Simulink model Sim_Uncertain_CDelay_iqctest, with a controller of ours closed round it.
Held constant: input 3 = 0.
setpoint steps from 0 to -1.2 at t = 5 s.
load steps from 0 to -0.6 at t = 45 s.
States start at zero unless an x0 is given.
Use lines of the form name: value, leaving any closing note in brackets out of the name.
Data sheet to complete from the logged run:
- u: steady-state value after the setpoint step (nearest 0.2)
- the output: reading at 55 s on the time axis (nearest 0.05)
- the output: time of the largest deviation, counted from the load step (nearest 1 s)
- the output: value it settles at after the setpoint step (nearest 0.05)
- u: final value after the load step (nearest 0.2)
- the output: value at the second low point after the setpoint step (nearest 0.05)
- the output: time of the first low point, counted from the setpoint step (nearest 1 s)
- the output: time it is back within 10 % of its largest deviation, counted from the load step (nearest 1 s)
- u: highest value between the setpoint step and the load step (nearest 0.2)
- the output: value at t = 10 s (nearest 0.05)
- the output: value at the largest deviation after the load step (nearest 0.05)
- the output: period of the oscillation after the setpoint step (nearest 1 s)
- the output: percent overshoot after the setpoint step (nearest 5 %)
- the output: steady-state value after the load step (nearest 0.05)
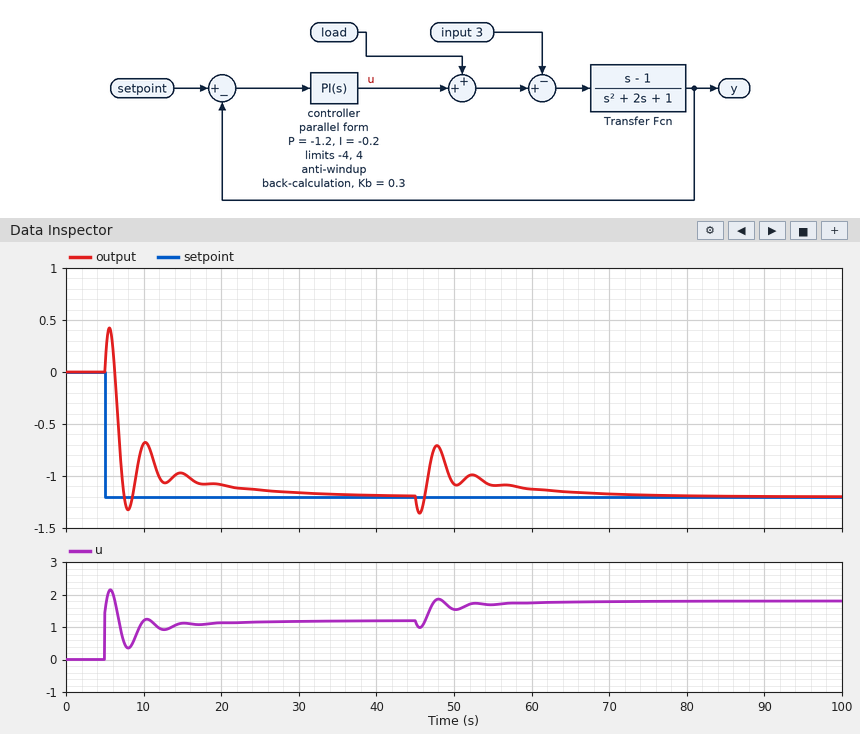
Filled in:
u: steady-state value after the setpoint step: 1.2
the output: reading at 55 s on the time axis: -1.10
the output: time of the largest deviation, counted from the load step: 3 s
the output: value it settles at after the setpoint step: -1.20
u: final value after the load step: 1.8
the output: value at the second low point after the setpoint step: -1.05
the output: time of the first low point, counted from the setpoint step: 3 s
the output: time it is back within 10 % of its largest deviation, counted from the load step: 19 s
u: highest value between the setpoint step and the load step: 2.2
the output: value at t = 10 s: -0.70
the output: value at the largest deviation after the load step: -0.70
the output: period of the oscillation after the setpoint step: 5 s
the output: percent overshoot after the setpoint step: 10 %
the output: steady-state value after the load step: -1.20
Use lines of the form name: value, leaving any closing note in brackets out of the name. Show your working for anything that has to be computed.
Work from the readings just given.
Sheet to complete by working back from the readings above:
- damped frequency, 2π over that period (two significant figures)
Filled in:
damped frequency, 2π over that period: 2π / 5 = 1.3 rad/s
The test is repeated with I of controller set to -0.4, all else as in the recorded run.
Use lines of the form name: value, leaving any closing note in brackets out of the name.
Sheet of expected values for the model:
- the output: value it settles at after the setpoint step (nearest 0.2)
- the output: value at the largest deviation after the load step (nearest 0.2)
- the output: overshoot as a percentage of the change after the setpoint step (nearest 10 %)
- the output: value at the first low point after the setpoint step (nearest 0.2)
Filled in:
the output: value it settles at after the setpoint step: -1.2
the output: value at the largest deviation after the load step: -0.6
the output: overshoot as a percentage of the change after the setpoint step: 40 %
the output: value at the first low point after the setpoint step: -1.6
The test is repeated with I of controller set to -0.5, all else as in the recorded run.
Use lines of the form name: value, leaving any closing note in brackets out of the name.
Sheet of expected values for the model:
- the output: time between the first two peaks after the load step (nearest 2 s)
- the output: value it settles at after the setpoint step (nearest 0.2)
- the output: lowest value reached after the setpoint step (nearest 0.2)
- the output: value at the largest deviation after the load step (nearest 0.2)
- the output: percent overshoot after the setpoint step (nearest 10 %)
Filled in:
the output: time between the first two peaks after the load step: 6 s
the output: value it settles at after the setpoint step: -1.2
the output: lowest value reached after the setpoint step: -1.8
the output: value at the largest deviation after the load step: -0.6
the output: percent overshoot after the setpoint step: 50 %
